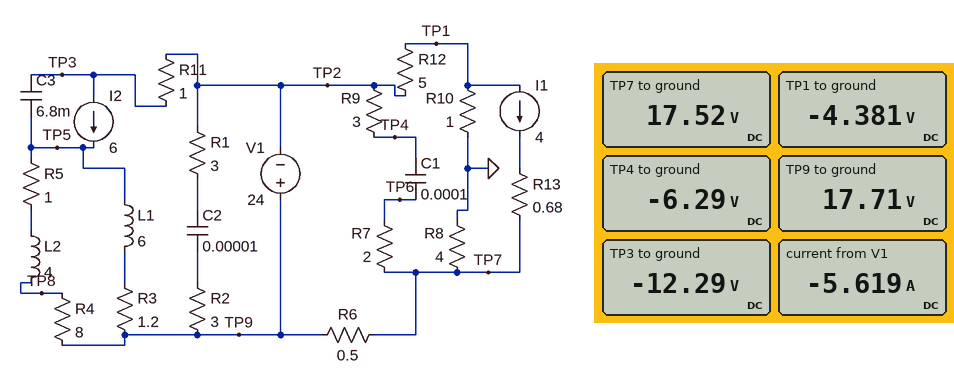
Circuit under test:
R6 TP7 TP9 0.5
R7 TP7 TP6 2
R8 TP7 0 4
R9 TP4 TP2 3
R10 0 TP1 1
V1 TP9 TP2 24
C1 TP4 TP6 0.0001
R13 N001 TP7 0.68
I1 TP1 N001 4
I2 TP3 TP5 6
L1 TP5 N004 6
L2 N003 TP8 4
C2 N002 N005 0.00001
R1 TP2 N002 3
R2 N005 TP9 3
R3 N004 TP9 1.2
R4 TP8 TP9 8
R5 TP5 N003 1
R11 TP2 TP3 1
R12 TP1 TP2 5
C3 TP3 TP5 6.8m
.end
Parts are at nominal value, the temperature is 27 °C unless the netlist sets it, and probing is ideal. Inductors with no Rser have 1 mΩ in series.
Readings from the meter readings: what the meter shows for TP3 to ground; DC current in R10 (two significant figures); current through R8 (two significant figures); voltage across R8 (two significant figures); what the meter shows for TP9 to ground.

-12.29 V
4.4 A
4.4 A
18 V
17.71 V
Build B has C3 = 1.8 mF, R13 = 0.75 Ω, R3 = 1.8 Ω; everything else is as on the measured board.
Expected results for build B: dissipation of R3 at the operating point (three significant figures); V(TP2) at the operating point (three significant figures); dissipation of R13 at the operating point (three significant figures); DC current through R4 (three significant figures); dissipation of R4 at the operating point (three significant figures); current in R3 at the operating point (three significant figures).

45.0 W
-6.29 V
12.0 W
1.00 A
8.01 W
5.00 A
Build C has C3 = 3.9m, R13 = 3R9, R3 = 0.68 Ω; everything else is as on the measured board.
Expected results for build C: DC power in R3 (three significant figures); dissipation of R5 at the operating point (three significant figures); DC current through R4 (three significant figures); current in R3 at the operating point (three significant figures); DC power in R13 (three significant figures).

21.2 W
178 mW
422 mA
5.58 A
62.4 W
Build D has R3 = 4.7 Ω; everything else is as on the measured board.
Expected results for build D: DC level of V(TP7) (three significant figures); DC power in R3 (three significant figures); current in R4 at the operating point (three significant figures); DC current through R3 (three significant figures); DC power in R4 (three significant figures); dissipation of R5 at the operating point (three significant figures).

17.5 V
73.0 W
2.06 A
3.94 A
33.9 W
4.24 W
